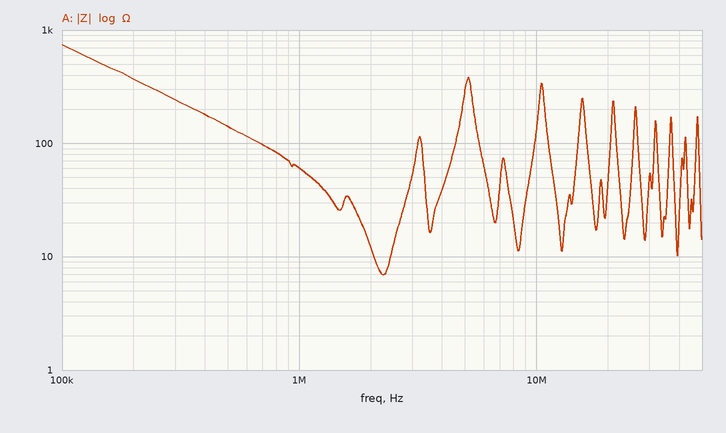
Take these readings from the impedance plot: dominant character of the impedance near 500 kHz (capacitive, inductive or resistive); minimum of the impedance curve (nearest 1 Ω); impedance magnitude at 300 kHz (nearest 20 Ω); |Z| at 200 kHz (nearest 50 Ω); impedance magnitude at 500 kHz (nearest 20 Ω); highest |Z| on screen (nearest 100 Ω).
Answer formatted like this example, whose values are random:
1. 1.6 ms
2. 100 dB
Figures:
1. capacitive
2. 7 Ω
3. 240 Ω
4. 350 Ω
5. 140 Ω
6. 700 Ω
